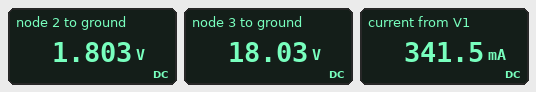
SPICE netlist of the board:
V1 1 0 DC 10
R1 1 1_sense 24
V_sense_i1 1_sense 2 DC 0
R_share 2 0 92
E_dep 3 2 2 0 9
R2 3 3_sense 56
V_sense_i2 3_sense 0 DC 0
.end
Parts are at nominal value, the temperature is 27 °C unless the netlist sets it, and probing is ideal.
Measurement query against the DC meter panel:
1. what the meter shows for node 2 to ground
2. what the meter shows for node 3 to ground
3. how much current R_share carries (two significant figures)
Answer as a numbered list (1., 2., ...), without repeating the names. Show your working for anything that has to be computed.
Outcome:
1. 1.803 V
2. 18.03 V
3. (1.803 V) / 92 Ω = 20 mA
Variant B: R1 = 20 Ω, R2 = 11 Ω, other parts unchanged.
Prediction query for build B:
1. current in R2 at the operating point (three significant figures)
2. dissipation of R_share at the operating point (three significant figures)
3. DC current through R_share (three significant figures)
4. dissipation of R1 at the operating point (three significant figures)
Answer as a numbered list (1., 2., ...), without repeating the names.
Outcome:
1. 469 mA
2. 2.89 mW
3. 5.60 mA
4. 4.50 W
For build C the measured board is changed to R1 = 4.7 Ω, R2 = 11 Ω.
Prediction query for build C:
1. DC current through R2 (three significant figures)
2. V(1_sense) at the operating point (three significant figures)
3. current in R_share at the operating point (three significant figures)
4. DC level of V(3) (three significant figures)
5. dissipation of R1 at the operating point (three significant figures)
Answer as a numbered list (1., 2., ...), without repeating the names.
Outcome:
1. 1.71 A
2. 1.88 V
3. 20.4 mA
4. 18.8 V
5. 14.0 W
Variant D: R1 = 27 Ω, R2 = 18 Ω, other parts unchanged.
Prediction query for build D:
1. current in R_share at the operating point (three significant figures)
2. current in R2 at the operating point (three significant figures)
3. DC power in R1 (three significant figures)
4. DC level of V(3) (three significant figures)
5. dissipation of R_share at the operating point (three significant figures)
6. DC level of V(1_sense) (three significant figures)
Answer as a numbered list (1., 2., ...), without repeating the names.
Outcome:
1. 6.67 mA
2. 341 mA
3. 3.26 W
4. 6.14 V
5. 4.09 mW
6. 614 mV
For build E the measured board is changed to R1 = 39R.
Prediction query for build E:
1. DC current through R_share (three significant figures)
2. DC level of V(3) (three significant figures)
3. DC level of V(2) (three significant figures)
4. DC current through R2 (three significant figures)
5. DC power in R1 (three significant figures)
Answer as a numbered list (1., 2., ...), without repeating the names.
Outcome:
1. 13.0 mA
2. 11.9 V
3. 1.19 V
4. 213 mA
5. 1.99 W
